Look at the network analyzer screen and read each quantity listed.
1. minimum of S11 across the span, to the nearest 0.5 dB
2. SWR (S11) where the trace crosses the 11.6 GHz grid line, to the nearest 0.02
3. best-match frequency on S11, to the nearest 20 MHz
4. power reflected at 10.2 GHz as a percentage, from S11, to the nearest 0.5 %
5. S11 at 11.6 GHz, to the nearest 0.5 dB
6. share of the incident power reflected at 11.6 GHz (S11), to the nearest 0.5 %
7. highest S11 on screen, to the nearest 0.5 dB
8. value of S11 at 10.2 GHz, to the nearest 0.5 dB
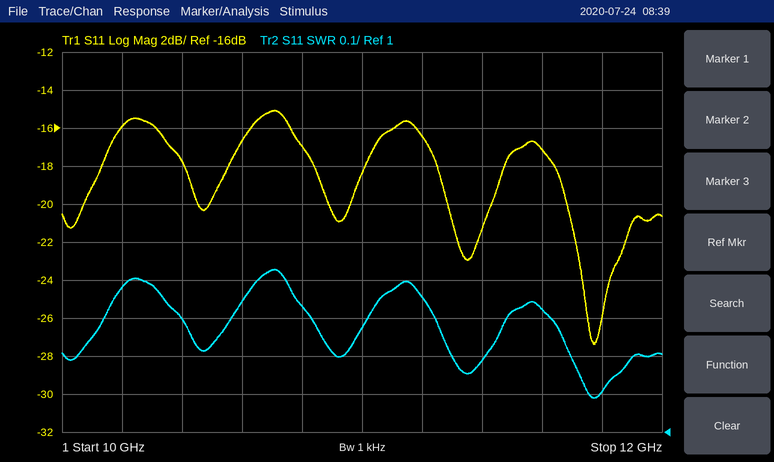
-27.5 dB
1.32
11.78 GHz
2.5 %
-17.0 dB
2.0 %
-15.0 dB
-16.0 dB
